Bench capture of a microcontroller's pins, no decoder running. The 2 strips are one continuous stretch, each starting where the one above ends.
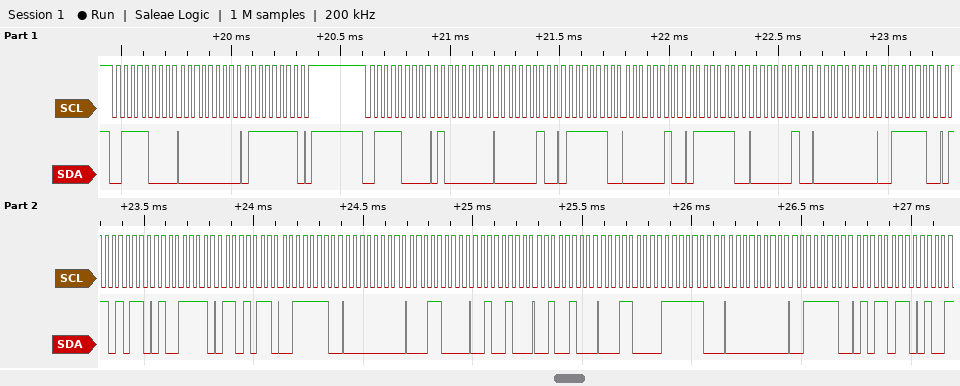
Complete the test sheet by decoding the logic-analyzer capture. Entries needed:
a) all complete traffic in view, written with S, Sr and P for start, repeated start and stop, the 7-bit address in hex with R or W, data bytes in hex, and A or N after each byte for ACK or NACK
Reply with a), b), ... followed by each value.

a) S 3CW A 00 A 7F A P S 3CW A 40 A 02 A 7E A 02 A 7E A 02 A 00 A 3E A 6B A 4F A 6B A 3E A 00 A 18 A 24 A 24 A 18 A FC A 00 A 3E A 5B A
